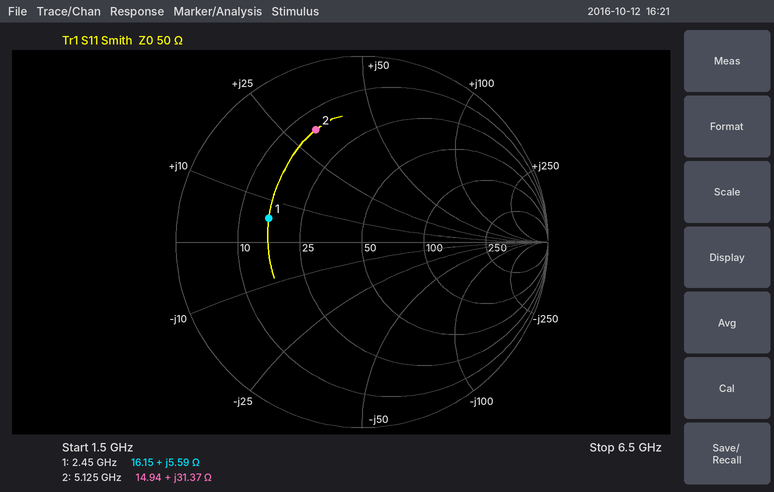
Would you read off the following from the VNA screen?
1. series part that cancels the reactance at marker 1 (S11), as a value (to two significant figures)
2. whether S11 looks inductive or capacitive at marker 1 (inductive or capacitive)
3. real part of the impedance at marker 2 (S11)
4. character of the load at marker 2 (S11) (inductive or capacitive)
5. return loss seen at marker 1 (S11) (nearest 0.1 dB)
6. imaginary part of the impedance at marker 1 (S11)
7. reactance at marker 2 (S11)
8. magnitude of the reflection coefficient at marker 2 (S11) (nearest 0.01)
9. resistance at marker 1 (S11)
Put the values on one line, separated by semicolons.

12 pF; inductive; 14.94 Ω; inductive; 5.7 dB; +5.59 Ω; +31.37 Ω; 0.65; 16.15 Ω
